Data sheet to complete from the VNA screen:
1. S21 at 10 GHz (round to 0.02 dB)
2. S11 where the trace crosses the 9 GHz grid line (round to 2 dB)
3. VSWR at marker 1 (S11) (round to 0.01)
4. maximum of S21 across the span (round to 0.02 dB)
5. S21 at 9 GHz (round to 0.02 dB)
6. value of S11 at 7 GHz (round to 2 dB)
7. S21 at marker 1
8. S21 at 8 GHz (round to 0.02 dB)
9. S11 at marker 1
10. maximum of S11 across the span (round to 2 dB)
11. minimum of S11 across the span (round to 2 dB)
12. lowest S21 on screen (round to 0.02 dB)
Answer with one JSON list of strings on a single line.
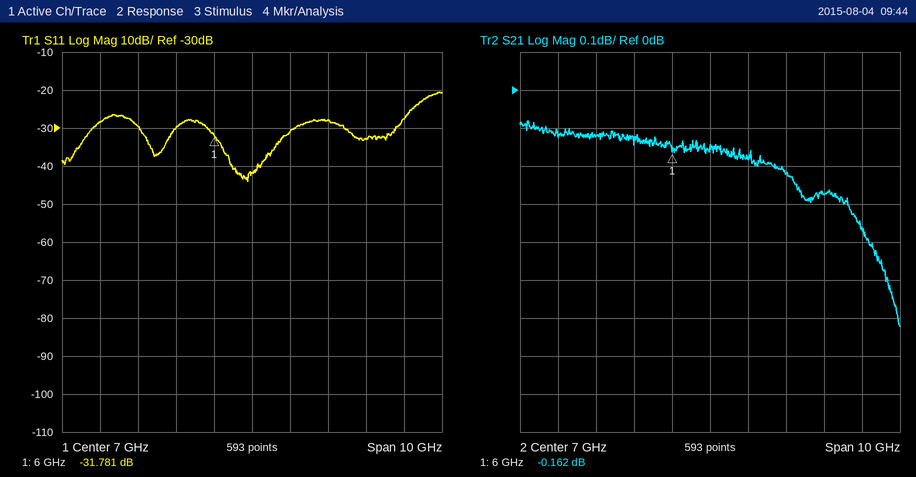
["-0.28 dB", "-28 dB", "1.05", "-0.08 dB", "-0.22 dB", "-42 dB", "-0.162 dB", "-0.18 dB", "-31.781 dB", "-20 dB", "-44 dB", "-0.62 dB"]
